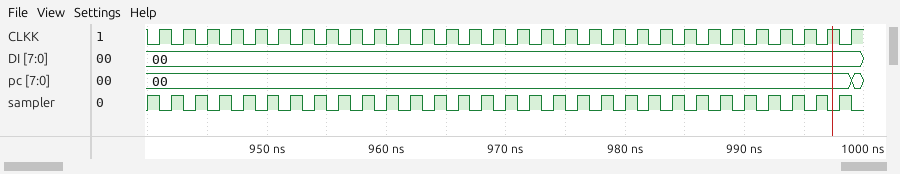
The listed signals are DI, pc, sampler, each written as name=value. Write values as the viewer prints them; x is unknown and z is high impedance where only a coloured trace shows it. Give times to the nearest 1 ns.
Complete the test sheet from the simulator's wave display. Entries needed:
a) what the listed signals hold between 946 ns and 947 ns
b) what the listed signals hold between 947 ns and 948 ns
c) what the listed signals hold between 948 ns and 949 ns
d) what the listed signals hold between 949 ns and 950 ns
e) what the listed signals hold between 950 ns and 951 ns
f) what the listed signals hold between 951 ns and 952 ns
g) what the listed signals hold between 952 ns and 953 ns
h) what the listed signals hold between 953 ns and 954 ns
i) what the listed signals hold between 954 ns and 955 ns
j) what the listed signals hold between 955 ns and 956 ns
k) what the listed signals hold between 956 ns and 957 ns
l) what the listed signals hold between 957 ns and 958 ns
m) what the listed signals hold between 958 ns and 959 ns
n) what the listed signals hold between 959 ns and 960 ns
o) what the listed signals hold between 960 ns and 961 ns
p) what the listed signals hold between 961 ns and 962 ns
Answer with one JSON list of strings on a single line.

["DI=00, pc=00, sampler=1", "DI=00, pc=00, sampler=0", "DI=00, pc=00, sampler=1", "DI=00, pc=00, sampler=0", "DI=00, pc=00, sampler=1", "DI=00, pc=00, sampler=0", "DI=00, pc=00, sampler=1", "DI=00, pc=00, sampler=0", "DI=00, pc=00, sampler=1", "DI=00, pc=00, sampler=0", "DI=00, pc=00, sampler=1", "DI=00, pc=00, sampler=0", "DI=00, pc=00, sampler=1", "DI=00, pc=00, sampler=0", "DI=00, pc=00, sampler=1", "DI=00, pc=00, sampler=0"]
